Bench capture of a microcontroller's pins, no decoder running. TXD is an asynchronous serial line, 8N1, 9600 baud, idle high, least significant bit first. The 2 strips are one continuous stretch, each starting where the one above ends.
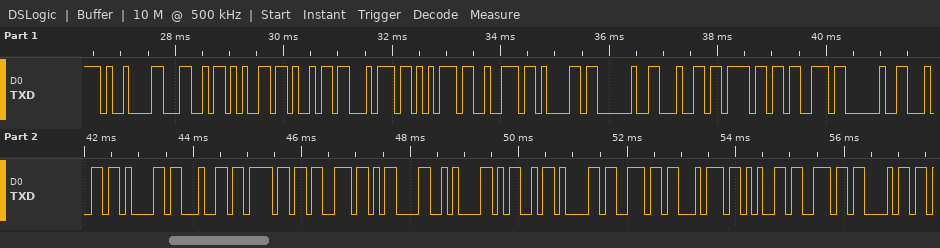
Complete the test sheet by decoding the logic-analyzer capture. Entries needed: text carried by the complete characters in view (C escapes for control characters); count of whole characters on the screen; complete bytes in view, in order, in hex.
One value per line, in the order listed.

"\tLeitura dos dados\r\nMantenh"
27
09 4C 65 69 74 75 72 61 20 64 6F 73 20 64 61 64 6F 73 0D 0A 4D 61 6E 74 65 6E 68
